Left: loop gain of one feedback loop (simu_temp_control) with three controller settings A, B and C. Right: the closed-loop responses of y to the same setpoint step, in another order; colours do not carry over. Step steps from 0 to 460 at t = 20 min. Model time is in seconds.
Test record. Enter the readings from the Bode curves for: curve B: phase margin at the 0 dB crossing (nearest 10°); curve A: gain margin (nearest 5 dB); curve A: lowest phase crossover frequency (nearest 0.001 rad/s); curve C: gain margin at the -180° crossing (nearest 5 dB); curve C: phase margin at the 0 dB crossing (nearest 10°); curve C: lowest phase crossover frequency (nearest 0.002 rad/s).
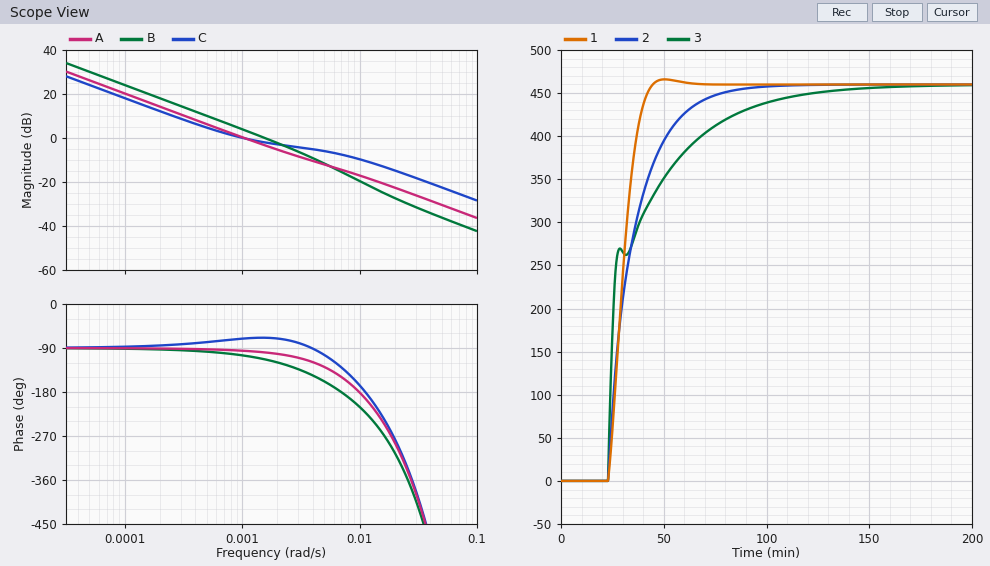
70°
15 dB
0.010 rad/s
10 dB
110°
0.012 rad/s
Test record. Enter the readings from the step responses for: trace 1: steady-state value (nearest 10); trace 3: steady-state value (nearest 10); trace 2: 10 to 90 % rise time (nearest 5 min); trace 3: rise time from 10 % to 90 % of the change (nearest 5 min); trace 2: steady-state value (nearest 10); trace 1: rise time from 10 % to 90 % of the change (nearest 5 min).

460
460
30 min
55 min
460
15 min
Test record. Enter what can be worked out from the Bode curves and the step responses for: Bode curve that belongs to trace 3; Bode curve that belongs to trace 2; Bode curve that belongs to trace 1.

C
A
B
